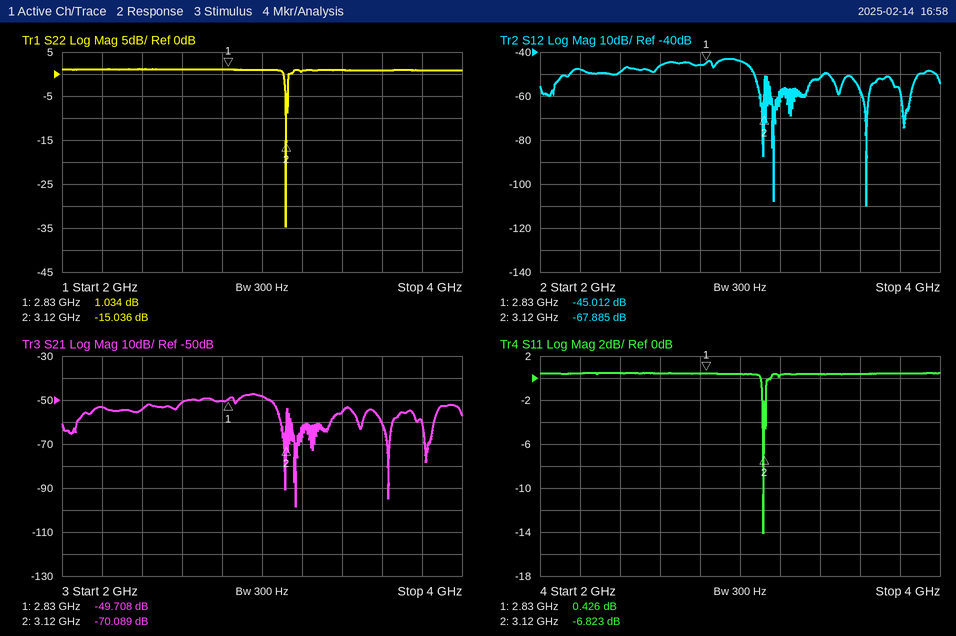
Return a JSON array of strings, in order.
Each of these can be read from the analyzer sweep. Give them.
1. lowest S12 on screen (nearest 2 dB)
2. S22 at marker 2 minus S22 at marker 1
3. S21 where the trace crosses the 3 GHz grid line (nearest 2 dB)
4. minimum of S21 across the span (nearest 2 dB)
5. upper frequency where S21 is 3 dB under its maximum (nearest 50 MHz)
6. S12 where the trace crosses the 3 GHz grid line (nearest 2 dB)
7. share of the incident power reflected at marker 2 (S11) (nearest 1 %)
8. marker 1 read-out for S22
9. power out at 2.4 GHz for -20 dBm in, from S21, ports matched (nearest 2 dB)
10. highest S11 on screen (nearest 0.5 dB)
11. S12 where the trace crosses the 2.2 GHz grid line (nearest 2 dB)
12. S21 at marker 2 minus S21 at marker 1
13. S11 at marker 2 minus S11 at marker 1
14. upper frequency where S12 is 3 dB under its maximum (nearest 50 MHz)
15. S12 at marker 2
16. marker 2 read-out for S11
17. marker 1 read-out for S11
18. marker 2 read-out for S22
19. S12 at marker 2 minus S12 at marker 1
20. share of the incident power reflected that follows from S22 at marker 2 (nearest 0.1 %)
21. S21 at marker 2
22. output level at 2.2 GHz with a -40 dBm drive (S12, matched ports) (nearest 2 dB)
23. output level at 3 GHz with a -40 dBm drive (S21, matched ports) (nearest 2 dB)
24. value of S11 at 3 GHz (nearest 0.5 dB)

["-110 dB", "-16.070 dB", "-48 dB", "-98 dB", "3.05 GHz", "-44 dB", "21 %", "1.034 dB", "-74 dBm", "0.5 dB", "-48 dB", "-20.381 dB", "-7.249 dB", "3.05 GHz", "-67.885 dB", "-6.823 dB", "0.426 dB", "-15.036 dB", "-22.873 dB", "3.1 %", "-70.089 dB", "-88 dBm", "-88 dBm", "0.5 dB"]
